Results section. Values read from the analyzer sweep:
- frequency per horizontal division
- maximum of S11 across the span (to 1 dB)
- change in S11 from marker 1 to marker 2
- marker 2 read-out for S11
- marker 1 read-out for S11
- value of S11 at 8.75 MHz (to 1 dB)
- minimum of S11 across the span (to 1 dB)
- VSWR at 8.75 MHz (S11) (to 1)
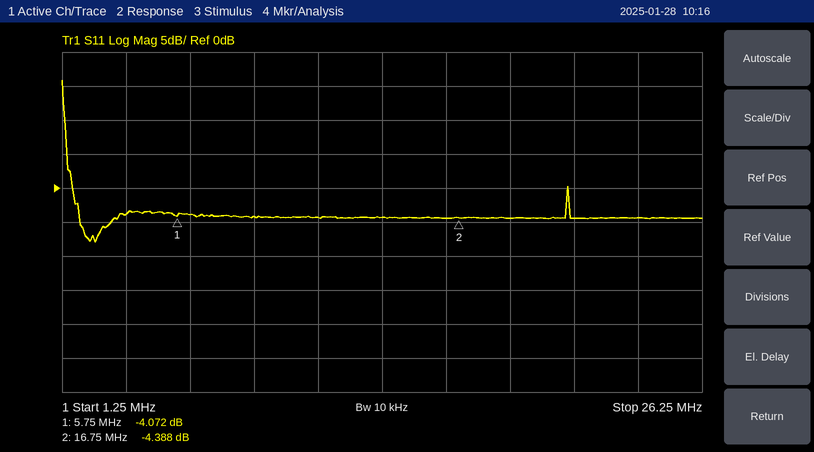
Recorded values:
2.5 MHz
16 dB
-0.316 dB
-4.388 dB
-4.072 dB
-4 dB
-8 dB
4
